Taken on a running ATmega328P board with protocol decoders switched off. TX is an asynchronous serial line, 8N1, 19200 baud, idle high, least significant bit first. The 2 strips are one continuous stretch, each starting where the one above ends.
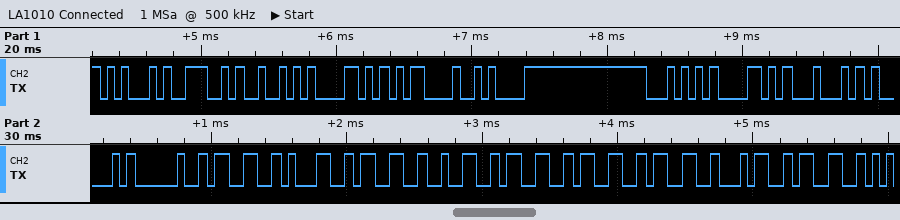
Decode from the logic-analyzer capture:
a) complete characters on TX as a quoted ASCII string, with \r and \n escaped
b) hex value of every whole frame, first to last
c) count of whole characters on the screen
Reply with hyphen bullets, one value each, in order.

- "ENRX\r\nTXDA 313233343"
- 45 4E 52 58 0D 0A 54 58 44 41 20 33 31 33 32 33 33 33 34 33
- 20
